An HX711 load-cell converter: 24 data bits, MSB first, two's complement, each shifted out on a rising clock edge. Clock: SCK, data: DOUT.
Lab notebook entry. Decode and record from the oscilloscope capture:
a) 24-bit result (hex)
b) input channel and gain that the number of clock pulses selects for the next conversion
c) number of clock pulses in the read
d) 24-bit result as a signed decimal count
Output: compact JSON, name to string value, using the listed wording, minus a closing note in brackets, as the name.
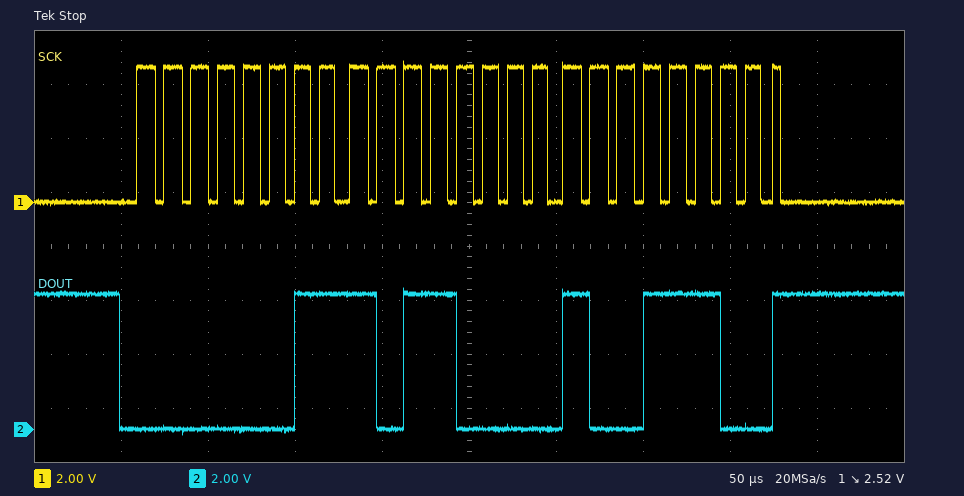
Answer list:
{"24-bit result": "0x03B09C", "input channel and gain that the number of clock pulses selects for the next conversion": "channel A, gain 128", "number of clock pulses in the read": "25", "24-bit result as a signed decimal count": "241820"}
